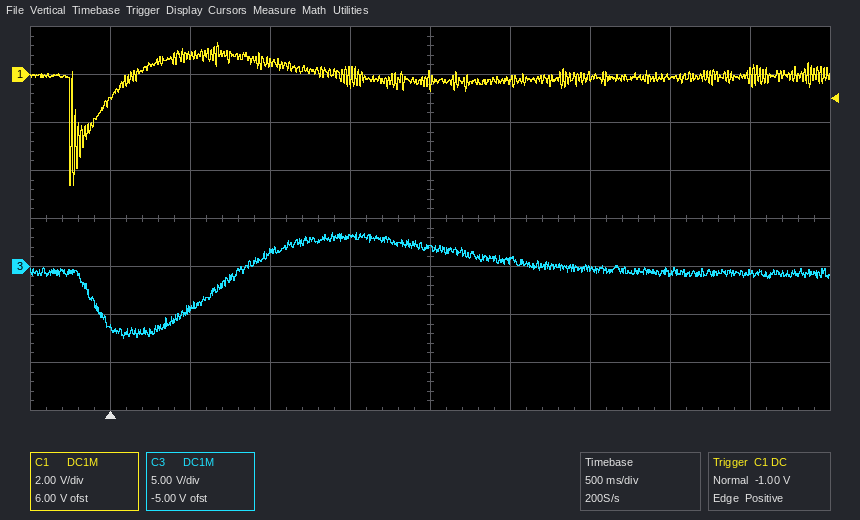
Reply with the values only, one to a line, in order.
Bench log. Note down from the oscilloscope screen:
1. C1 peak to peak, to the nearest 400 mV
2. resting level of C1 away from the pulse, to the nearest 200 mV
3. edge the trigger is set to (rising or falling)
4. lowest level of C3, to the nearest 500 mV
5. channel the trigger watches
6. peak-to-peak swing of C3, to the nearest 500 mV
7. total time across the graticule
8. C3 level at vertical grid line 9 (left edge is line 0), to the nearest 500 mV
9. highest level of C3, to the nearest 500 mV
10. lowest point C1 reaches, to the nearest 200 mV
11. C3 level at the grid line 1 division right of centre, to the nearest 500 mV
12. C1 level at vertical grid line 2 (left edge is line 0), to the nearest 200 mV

6.0 V
-200 mV
rising
-7.5 V
C1
11.0 V
5 s
-500 mV
3.5 V
-4.6 V
500 mV
800 mV
